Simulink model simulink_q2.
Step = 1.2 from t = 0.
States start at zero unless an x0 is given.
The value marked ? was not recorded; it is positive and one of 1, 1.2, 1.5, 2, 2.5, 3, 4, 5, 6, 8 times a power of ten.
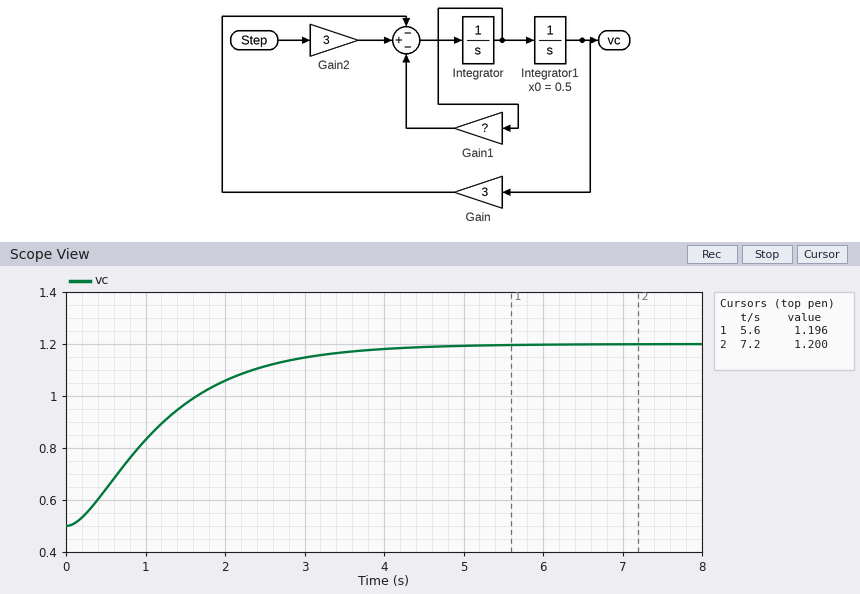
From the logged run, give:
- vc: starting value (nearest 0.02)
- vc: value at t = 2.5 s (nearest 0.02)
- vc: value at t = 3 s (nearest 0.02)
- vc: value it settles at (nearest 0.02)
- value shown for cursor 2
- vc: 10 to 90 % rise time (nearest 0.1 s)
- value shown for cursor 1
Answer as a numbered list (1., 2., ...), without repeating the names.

1. 0.50
2. 1.12
3. 1.14
4. 1.20
5. 1.200
6. 2.4 s
7. 1.196
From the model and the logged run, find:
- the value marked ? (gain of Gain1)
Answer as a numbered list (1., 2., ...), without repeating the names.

1. 4
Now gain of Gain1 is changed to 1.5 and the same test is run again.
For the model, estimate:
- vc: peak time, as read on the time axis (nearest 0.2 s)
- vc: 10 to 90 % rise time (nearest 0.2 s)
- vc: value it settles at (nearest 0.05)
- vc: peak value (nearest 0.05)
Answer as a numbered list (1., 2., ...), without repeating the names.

1. 2.0 s
2. 0.8 s
3. 1.20
4. 1.35
